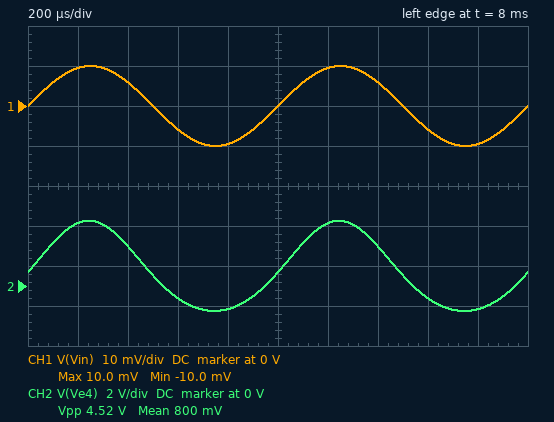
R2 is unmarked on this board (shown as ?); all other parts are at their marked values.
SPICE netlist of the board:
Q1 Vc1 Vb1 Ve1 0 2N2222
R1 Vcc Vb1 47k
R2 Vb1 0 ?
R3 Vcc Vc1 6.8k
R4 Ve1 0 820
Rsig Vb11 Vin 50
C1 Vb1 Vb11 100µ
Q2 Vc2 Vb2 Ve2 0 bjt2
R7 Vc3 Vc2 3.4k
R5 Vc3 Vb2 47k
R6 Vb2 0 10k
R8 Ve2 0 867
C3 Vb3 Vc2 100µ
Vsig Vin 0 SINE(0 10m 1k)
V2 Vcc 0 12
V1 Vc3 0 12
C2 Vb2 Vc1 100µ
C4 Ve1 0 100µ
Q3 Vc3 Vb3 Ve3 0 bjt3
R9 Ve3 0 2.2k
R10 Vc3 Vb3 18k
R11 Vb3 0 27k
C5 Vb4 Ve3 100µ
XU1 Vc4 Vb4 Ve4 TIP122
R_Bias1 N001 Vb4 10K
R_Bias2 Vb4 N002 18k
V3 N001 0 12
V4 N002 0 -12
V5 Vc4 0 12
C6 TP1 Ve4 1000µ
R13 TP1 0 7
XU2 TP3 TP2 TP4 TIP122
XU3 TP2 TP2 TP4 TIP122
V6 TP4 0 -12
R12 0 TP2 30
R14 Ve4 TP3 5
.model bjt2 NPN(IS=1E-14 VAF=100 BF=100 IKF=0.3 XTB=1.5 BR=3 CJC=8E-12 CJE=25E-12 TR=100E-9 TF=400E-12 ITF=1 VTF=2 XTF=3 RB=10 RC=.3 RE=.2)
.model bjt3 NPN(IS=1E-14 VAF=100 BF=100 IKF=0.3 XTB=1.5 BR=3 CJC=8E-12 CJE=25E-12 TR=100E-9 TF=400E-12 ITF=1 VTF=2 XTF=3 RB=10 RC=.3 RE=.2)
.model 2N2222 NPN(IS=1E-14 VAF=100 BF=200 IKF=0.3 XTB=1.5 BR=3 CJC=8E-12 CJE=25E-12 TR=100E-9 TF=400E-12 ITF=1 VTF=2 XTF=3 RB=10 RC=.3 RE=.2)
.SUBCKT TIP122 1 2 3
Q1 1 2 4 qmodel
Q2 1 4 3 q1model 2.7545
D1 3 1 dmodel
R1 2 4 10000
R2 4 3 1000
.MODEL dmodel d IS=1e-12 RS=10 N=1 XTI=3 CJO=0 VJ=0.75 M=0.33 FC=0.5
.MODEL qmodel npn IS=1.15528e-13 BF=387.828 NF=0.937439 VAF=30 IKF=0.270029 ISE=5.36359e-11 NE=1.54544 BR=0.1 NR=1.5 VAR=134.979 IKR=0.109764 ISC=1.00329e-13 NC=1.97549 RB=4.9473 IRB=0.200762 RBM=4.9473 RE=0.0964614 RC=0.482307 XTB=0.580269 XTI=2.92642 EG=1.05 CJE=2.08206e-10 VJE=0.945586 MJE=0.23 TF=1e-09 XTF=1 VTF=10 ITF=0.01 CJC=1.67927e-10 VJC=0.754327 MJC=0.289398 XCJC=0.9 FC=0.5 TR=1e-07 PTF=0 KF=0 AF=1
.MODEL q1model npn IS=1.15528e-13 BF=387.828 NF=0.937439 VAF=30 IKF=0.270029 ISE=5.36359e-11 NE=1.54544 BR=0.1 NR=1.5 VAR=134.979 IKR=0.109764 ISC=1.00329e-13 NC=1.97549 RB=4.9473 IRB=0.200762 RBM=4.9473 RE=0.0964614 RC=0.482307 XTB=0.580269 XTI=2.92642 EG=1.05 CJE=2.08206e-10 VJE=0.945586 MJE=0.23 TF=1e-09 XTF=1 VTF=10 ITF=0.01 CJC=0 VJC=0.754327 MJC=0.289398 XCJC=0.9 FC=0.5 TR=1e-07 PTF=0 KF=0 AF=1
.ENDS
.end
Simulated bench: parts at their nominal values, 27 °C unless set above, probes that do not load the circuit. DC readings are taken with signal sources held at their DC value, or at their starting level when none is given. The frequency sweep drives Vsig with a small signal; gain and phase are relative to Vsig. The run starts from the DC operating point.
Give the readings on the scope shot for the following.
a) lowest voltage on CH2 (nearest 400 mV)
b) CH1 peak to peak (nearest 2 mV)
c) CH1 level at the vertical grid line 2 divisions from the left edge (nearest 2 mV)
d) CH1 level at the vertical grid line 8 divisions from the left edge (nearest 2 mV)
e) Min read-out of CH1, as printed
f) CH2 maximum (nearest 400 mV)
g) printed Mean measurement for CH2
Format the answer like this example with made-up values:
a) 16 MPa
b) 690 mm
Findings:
a) -1.2 V
b) 20 mV
c) 6 mV
d) -6 mV
e) -10.0 mV
f) 3.2 V
g) 800 mV
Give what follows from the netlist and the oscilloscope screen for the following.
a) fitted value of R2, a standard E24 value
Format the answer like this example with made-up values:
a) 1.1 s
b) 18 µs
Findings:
a) 5.1 kΩ
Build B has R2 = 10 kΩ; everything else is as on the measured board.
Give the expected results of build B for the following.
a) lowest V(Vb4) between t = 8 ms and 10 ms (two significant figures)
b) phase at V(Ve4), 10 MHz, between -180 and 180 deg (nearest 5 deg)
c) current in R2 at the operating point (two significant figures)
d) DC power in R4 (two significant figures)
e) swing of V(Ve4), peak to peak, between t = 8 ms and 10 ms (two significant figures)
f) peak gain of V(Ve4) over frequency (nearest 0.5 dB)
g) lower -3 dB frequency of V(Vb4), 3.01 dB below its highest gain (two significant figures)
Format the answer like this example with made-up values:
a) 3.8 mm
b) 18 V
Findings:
a) -1.1 V
b) 155 deg
c) 200 µA
d) 2.0 mW
e) 3.3 V
f) 34.5 dB
g) 33 Hz
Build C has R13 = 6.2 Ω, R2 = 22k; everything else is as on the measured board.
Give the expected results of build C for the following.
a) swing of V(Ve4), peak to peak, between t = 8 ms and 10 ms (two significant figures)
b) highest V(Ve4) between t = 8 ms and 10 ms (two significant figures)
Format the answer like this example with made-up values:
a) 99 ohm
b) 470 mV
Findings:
a) 120 mV
b) 820 mV
